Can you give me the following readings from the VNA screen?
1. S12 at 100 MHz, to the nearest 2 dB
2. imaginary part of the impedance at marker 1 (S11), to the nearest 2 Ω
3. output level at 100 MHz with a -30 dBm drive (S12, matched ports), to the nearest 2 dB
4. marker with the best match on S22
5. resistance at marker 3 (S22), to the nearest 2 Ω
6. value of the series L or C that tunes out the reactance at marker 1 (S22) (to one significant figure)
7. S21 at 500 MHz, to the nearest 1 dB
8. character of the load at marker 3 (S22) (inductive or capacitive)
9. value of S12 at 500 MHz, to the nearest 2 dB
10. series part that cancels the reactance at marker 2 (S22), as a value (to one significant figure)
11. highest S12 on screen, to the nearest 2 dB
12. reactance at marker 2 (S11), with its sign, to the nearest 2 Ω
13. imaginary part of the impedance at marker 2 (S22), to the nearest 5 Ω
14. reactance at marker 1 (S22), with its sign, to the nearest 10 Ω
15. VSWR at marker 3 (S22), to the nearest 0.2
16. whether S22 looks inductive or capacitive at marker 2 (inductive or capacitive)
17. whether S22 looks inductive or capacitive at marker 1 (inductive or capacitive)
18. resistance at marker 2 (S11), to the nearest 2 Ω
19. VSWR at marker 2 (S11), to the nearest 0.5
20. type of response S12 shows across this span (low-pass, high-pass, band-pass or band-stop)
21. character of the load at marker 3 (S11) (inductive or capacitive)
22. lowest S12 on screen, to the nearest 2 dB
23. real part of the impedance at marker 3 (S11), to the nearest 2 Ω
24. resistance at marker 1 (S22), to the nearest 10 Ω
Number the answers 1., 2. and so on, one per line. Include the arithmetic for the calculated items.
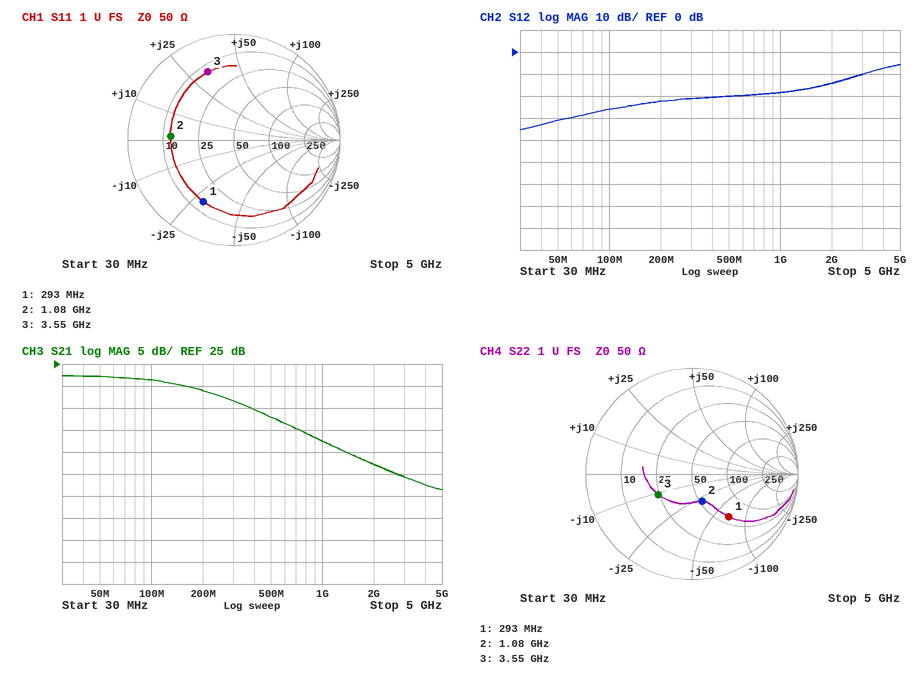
1. -26 dB
2. -30 Ω
3. -30 dBm + (-26 dB) = -56 dBm
4. marker 2
5. 24 Ω
6. L = 70 Ω/(2π × 293 MHz) ≈ 38.0 nH, so 40 nH to one significant figure
7. 13 dB
8. capacitive
9. -20 dB
10. L = 30 Ω/(2π × 1.08 GHz) ≈ 4 nH
11. -6 dB
12. +2 Ω
13. -30 Ω
14. -70 Ω
15. 2.2
16. capacitive
17. capacitive
18. 12 Ω
19. 4.0
20. high-pass
21. inductive
22. -36 dB
23. 14 Ω
24. 60 Ω
